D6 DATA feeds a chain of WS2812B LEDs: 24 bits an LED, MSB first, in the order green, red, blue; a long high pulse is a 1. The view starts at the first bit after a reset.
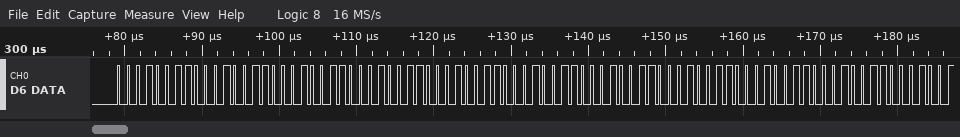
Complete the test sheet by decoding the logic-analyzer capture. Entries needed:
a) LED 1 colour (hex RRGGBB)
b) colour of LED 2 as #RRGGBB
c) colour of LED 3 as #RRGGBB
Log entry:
#131313
#131313
#131313
